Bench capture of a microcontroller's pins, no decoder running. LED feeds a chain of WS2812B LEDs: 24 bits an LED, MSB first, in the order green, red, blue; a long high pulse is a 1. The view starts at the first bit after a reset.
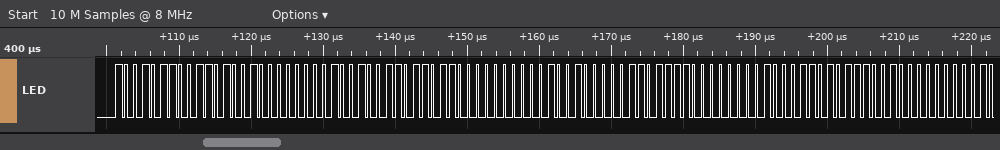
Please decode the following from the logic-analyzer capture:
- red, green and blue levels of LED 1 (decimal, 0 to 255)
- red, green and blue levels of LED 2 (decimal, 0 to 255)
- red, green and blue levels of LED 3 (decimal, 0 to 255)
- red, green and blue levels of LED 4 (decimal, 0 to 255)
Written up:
105, 150, 0
108, 147, 0
111, 144, 0
114, 141, 0
